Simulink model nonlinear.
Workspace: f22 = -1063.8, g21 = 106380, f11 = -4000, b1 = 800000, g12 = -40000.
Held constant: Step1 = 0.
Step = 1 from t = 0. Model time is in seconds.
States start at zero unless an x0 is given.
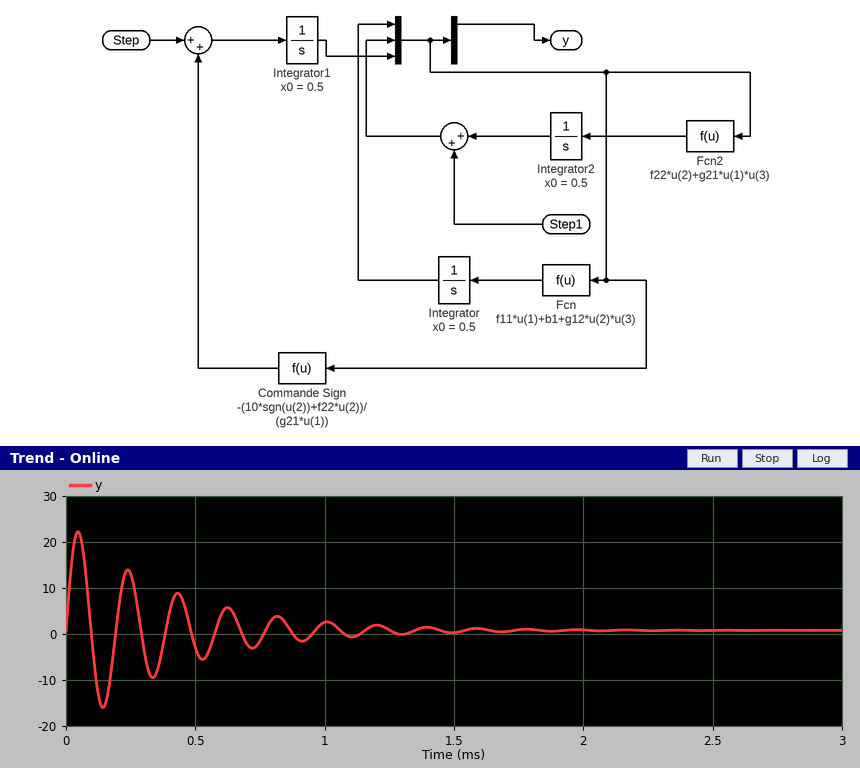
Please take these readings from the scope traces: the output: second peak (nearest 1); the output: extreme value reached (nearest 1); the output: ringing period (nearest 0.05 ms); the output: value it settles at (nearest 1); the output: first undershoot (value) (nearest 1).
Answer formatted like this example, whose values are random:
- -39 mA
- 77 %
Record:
- 14
- 22
- 0.20 ms
- 1
- -16
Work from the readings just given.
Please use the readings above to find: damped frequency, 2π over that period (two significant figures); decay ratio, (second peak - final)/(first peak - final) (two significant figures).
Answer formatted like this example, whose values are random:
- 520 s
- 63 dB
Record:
- 31 rad/ms
- 0.62
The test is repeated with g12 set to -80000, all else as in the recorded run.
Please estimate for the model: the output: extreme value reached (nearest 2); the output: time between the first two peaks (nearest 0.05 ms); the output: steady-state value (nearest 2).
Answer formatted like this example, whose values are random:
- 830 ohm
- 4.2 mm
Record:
- 16
- 0.15 ms
- 0
